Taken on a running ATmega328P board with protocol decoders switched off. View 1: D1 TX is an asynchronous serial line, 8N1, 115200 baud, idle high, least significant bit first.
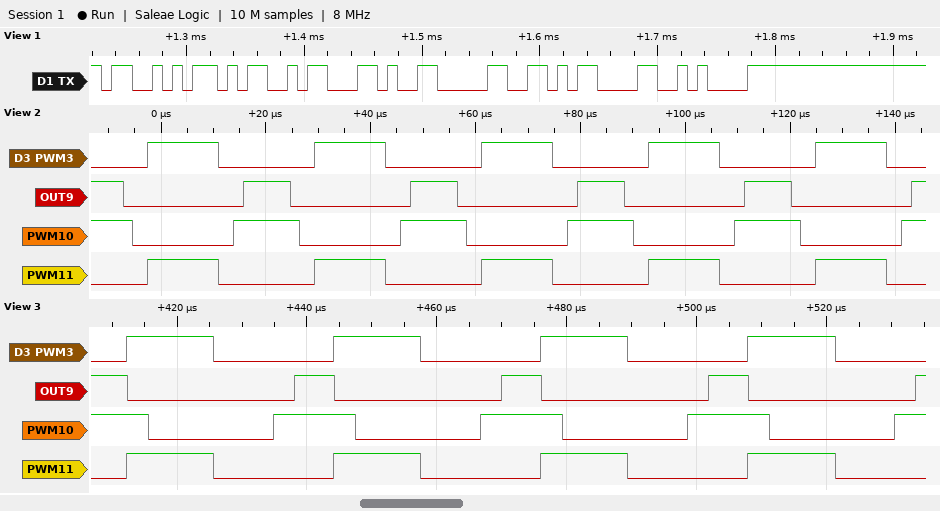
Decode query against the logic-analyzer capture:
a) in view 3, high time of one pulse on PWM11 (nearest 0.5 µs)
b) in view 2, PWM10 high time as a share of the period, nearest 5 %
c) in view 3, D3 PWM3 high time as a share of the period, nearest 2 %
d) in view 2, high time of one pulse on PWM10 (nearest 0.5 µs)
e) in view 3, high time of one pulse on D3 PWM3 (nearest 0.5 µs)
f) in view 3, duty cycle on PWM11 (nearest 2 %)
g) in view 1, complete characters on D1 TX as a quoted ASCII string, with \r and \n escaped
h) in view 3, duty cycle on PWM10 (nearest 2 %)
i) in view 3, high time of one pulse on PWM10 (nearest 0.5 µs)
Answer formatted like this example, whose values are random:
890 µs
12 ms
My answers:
13.5 µs
40 %
42 %
12.5 µs
13.5 µs
42 %
"SM,0\r\n"
40 %
12.5 µs
